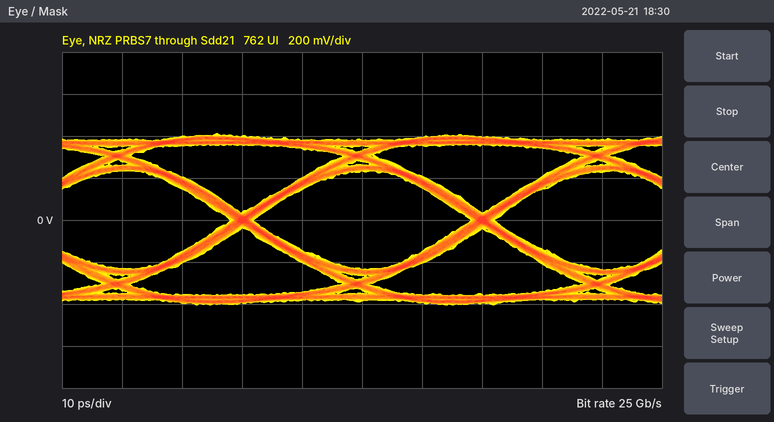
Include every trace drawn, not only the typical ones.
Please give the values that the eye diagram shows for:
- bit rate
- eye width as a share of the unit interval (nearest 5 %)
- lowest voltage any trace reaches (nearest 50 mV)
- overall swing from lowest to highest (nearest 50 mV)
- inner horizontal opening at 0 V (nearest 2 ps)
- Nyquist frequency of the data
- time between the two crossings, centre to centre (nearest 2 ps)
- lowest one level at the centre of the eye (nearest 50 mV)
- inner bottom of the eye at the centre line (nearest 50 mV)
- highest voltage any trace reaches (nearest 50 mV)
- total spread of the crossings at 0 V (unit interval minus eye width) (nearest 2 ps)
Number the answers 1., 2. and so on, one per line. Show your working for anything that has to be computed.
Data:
1. 25 Gb/s
2. 36 ps / 40 ps ≈ 90 %
3. -400 mV
4. 800 mV
5. 36 ps
6. 12.5 GHz
7. 40 ps
8. 250 mV
9. -250 mV
10. 400 mV
11. 4 ps
